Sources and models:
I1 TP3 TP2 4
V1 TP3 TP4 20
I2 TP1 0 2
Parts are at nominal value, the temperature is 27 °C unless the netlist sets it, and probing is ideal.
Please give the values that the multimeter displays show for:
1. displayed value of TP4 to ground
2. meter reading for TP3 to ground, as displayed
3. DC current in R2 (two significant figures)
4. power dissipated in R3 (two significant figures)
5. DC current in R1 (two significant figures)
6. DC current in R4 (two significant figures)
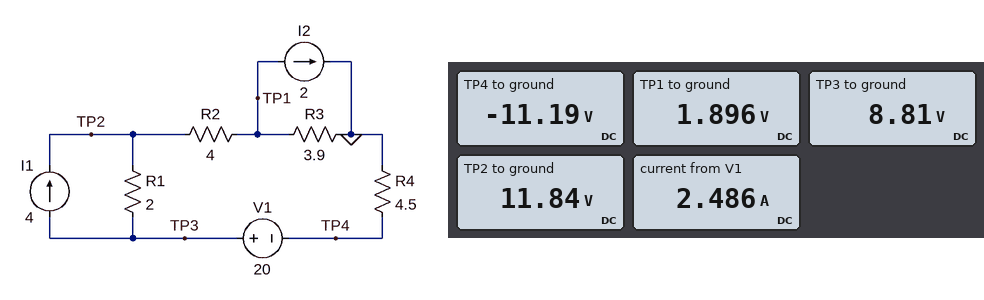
-11.19 V
8.81 V
2.5 A
920 mW
1.5 A
2.5 A
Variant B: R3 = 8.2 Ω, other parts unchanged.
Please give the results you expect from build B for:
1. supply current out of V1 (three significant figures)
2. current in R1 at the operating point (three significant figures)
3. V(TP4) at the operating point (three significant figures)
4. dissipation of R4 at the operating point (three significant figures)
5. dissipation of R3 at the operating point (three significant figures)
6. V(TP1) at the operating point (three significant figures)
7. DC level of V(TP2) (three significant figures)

2.37 A
1.63 A
-10.7 V
25.4 W
1.15 W
3.07 V
12.6 V
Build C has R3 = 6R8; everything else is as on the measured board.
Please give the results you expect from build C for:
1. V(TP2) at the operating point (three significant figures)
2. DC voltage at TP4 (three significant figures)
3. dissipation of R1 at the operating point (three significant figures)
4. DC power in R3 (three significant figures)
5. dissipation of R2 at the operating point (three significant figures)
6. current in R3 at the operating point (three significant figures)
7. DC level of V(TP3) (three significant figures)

12.4 V
-10.8 V
5.09 W
1.11 W
23.1 W
405 mA
9.18 V
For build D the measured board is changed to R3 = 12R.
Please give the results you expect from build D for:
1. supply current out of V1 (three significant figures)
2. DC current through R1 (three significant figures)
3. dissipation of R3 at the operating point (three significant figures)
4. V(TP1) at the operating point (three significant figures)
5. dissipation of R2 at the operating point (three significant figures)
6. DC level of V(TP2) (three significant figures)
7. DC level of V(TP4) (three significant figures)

2.31 A
1.69 A
1.16 W
3.73 V
21.4 W
13.0 V
-10.4 V
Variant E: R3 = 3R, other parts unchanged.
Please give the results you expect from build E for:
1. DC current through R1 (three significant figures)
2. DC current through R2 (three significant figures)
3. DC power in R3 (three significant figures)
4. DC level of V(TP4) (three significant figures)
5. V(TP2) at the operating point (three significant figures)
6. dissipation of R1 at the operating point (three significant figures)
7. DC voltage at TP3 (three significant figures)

1.48 A
2.52 A
807 mW
-11.3 V
11.6 V
4.39 W
8.67 V
